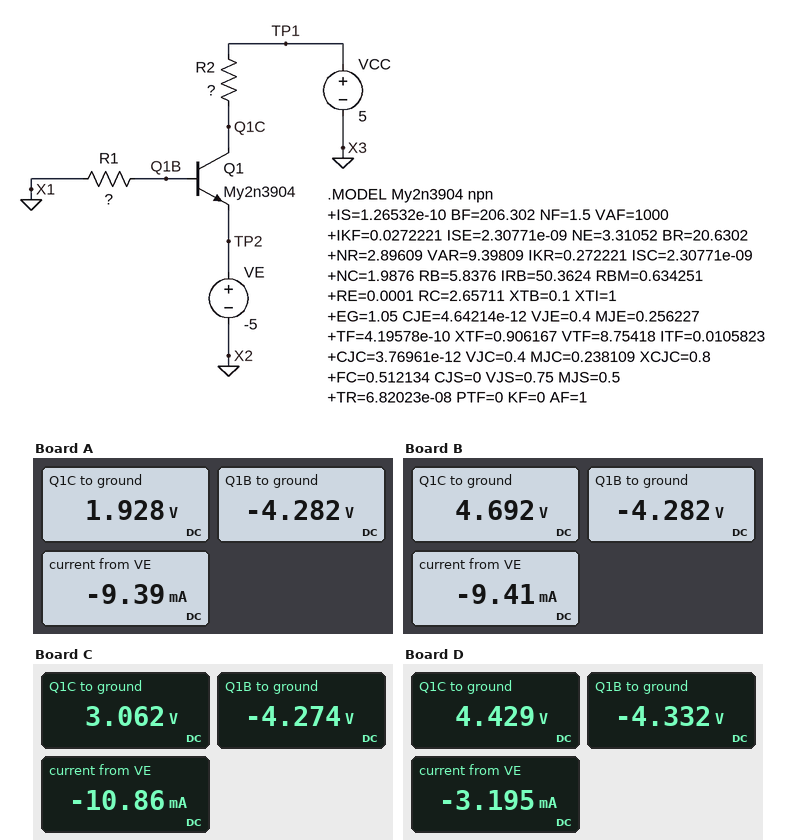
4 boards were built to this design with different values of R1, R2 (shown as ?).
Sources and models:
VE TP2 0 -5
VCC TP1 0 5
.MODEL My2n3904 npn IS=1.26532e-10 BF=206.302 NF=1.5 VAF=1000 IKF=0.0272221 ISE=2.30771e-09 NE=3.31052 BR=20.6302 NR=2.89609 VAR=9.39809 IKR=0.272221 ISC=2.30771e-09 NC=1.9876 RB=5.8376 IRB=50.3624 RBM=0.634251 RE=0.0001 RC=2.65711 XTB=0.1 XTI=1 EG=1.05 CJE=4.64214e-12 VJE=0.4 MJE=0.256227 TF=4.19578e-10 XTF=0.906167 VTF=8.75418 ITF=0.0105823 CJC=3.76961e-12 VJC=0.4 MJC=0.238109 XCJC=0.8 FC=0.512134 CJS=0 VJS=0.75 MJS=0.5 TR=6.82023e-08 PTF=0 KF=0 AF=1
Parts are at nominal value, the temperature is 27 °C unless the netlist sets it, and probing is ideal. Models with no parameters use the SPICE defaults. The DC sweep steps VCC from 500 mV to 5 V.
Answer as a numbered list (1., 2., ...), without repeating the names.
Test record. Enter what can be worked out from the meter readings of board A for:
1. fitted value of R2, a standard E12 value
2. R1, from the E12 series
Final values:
1. 330 Ω
2. 56 kΩ
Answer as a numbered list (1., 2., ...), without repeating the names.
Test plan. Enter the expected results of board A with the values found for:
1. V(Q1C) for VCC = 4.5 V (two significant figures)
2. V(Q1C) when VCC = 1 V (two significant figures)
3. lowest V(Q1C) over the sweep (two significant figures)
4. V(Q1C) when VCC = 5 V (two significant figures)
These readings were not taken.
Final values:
1. 1.4 V
2. -2.1 V
3. -2.6 V
4. 1.9 V
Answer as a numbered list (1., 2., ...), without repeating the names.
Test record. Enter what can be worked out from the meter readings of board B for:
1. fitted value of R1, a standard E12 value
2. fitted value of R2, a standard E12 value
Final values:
1. 56 kΩ
2. 33 Ω
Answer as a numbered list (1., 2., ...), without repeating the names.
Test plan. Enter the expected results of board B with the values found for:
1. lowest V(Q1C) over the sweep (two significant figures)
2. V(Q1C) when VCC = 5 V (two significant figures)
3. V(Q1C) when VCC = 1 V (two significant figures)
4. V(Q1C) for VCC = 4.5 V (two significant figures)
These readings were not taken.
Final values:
1. 190 mV
2. 4.7 V
3. 690 mV
4. 4.2 V
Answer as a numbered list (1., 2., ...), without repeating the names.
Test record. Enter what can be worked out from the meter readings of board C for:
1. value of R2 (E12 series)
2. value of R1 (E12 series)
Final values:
1. 180 Ω
2. 47 kΩ
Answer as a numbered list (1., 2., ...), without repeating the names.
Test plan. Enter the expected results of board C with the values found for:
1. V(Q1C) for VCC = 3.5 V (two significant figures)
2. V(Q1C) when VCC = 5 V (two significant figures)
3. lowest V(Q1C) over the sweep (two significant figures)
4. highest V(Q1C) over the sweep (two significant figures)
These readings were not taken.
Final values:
1. 1.6 V
2. 3.1 V
3. -1.4 V
4. 3.1 V
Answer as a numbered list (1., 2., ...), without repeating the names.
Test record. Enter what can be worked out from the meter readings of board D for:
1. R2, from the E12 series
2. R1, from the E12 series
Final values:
1. 180 Ω
2. 180 kΩ
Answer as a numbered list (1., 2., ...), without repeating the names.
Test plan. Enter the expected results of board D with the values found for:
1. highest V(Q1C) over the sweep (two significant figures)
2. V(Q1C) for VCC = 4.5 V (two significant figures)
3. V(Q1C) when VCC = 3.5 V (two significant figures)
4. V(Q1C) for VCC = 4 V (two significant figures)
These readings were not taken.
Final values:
1. 4.4 V
2. 3.9 V
3. 2.9 V
4. 3.4 V
